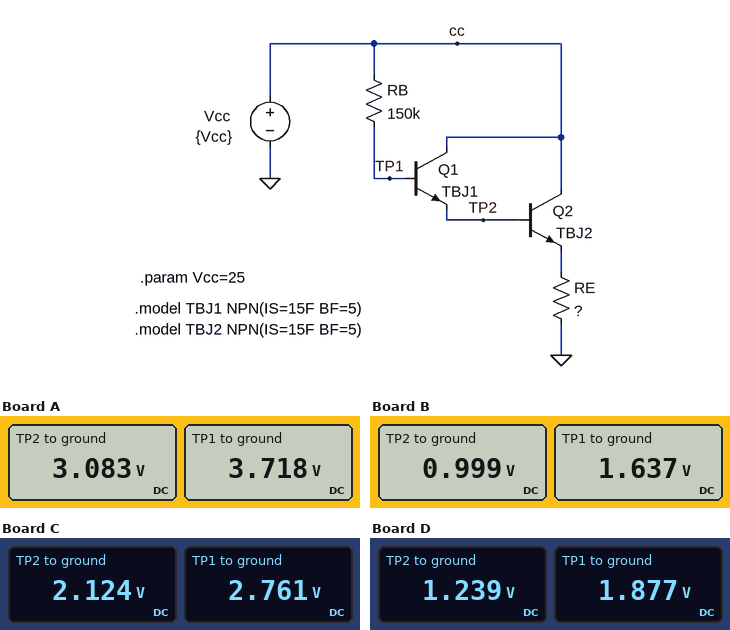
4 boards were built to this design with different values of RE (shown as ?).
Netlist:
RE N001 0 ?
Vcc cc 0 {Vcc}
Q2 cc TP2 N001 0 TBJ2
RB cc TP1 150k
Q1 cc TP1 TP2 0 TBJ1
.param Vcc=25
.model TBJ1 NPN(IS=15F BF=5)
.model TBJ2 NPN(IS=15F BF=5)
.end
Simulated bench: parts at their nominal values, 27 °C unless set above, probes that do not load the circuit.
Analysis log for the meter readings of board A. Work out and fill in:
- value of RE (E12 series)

470 Ω
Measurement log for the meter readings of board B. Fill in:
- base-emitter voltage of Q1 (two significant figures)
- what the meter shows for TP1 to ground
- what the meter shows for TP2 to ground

640 mV
1.637 V
0.999 V
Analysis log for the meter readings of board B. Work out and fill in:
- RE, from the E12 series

56 Ω
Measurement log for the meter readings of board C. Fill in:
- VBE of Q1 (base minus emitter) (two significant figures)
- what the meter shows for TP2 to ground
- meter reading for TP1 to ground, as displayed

640 mV
2.124 V
2.761 V
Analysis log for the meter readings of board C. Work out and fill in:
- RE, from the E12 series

270 Ω
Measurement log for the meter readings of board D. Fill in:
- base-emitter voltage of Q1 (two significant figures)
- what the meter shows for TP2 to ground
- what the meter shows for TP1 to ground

640 mV
1.239 V
1.877 V
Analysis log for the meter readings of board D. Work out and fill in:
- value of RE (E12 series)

100 Ω
